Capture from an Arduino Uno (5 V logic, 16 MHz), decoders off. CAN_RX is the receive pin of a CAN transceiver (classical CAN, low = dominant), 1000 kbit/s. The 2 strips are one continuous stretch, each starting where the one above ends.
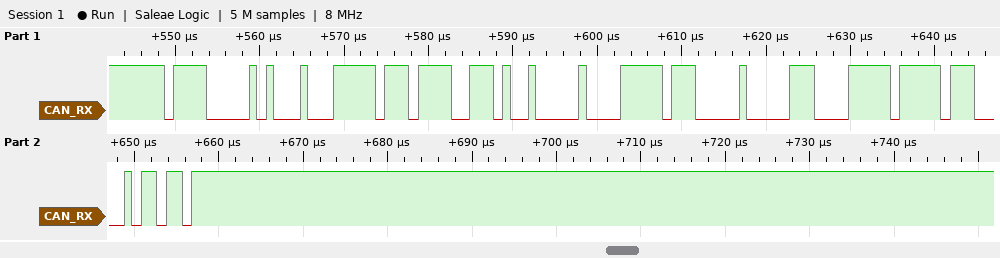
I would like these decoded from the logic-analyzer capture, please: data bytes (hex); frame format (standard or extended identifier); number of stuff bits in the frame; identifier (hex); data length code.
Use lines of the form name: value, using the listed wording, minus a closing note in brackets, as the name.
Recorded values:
data bytes: FF 79 D2 00 FF 00 30 FF
frame format: standard
number of stuff bits in the frame: 8
identifier: 0x781
data length code: 8
